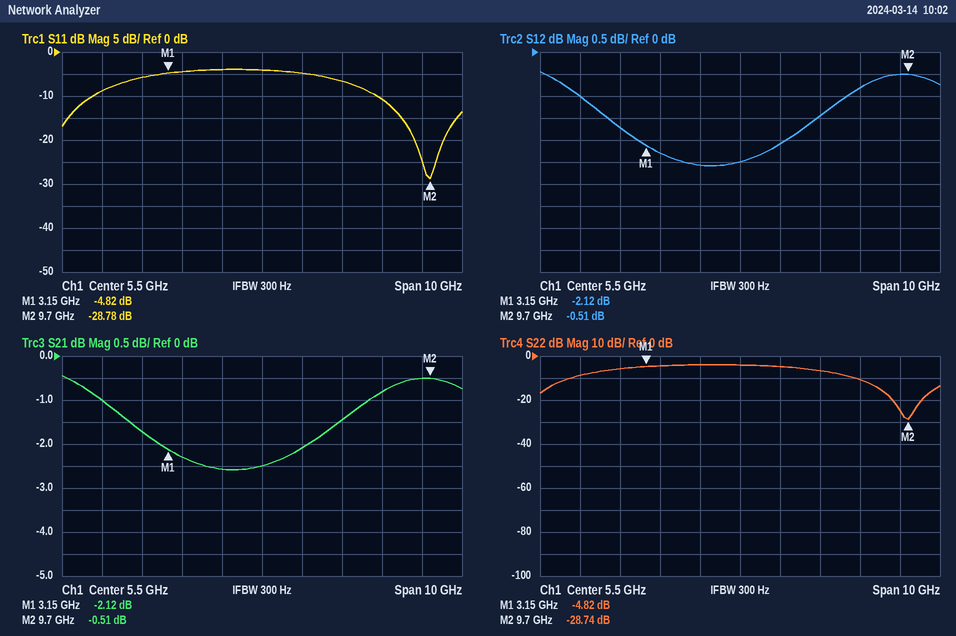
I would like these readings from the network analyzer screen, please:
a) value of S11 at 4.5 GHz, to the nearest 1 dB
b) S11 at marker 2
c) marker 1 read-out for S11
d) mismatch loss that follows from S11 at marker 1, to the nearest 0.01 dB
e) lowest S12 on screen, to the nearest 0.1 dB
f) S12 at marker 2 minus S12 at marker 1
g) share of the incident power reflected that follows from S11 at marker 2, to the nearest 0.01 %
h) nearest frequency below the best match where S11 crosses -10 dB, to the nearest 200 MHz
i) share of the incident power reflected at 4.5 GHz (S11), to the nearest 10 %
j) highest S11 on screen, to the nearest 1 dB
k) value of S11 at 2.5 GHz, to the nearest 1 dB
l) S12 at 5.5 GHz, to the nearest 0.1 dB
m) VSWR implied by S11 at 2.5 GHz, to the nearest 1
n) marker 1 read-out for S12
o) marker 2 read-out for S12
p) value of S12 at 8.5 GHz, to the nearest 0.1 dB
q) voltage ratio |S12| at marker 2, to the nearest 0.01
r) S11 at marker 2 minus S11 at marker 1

-4 dB
-28.78 dB
-4.82 dB
1.74 dB
-2.6 dB
1.61 dB
0.13 %
8.4 GHz
40 %
-4 dB
-6 dB
-2.5 dB
3
-2.12 dB
-0.51 dB
-0.8 dB
0.94
-23.96 dB
